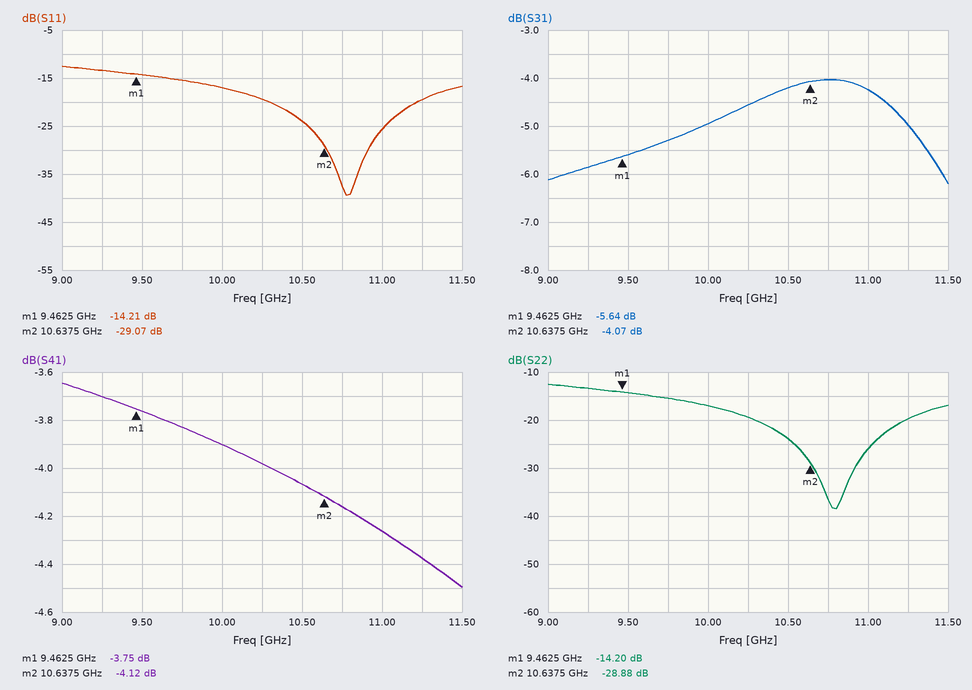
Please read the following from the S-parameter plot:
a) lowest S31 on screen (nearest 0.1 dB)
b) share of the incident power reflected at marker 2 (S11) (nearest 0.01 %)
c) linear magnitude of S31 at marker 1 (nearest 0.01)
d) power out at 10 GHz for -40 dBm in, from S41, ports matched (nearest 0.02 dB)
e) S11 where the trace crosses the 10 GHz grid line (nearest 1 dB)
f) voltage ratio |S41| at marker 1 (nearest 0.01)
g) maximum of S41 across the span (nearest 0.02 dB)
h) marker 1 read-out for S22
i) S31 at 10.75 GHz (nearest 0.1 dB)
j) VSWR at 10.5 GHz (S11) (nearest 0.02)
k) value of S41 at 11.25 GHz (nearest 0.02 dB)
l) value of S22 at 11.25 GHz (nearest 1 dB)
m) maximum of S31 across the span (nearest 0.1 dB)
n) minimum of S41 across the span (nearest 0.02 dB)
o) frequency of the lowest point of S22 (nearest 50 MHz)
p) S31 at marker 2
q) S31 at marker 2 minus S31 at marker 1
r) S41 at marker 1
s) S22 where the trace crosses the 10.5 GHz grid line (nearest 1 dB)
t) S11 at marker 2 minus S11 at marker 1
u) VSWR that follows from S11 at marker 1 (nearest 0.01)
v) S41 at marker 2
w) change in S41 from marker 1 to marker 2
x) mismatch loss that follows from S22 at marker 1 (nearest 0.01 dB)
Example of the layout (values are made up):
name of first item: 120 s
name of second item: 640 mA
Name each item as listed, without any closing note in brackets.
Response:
lowest S31 on screen: -6.2 dB
share of the incident power reflected at marker 2 (S11): 0.12 %
linear magnitude of S31 at marker 1: 0.52
power out at 10 GHz for -40 dBm in, from S41, ports matched: -43.90 dBm
S11 where the trace crosses the 10 GHz grid line: -17 dB
voltage ratio |S41| at marker 1: 0.65
maximum of S41 across the span: -3.64 dB
marker 1 read-out for S22: -14.20 dB
S31 at 10.75 GHz: -4.0 dB
VSWR at 10.5 GHz (S11): 1.14
value of S41 at 11.25 GHz: -4.38 dB
value of S22 at 11.25 GHz: -20 dB
maximum of S31 across the span: -4.0 dB
minimum of S41 across the span: -4.50 dB
frequency of the lowest point of S22: 10.80 GHz
S31 at marker 2: -4.07 dB
S31 at marker 2 minus S31 at marker 1: 1.57 dB
S41 at marker 1: -3.75 dB
S22 where the trace crosses the 10.5 GHz grid line: -24 dB
S11 at marker 2 minus S11 at marker 1: -14.86 dB
VSWR that follows from S11 at marker 1: 1.48
S41 at marker 2: -4.12 dB
change in S41 from marker 1 to marker 2: -0.37 dB
mismatch loss that follows from S22 at marker 1: 0.17 dB
